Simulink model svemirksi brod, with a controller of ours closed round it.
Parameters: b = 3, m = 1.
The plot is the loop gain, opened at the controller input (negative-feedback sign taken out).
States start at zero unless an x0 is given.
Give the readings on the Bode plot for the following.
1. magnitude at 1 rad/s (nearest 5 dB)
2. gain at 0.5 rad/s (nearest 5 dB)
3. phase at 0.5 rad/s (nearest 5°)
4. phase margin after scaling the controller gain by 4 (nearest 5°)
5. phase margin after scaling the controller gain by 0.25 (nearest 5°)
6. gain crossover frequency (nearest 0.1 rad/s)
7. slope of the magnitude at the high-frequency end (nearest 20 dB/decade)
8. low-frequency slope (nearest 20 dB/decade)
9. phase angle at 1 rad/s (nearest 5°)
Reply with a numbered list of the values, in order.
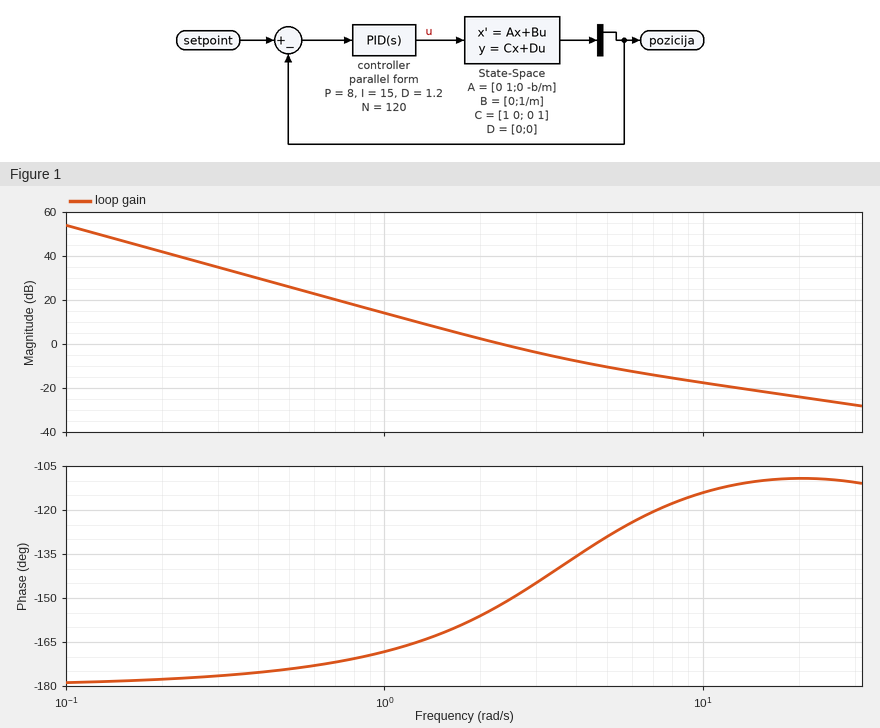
1. 15 dB
2. 25 dB
3. -175°
4. 55°
5. 15°
6. 2.3 rad/s
7. -20 dB/decade
8. -40 dB/decade
9. -170°
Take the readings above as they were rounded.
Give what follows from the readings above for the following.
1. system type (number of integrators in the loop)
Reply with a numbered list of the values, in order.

1. 2
